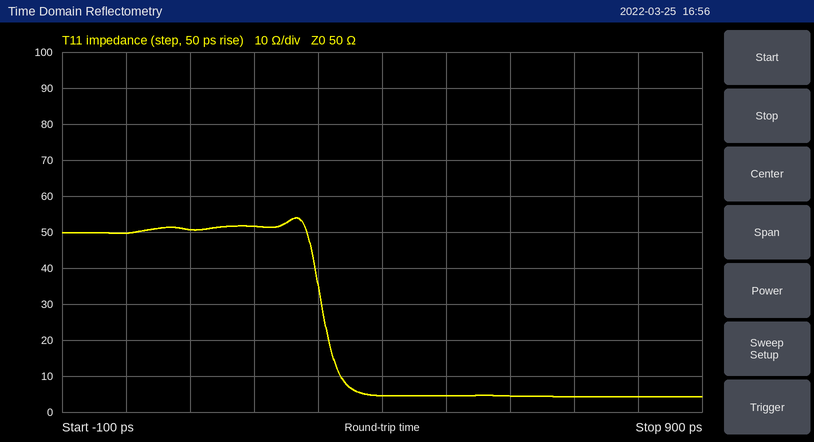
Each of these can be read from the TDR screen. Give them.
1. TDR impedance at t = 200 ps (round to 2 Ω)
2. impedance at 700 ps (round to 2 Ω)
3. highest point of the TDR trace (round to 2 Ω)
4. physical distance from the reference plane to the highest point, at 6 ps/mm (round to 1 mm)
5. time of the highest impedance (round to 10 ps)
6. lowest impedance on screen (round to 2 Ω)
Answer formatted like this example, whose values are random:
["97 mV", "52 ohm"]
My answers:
["52 Ω", "4 Ω", "54 Ω", "22 mm", "270 ps", "4 Ω"]
